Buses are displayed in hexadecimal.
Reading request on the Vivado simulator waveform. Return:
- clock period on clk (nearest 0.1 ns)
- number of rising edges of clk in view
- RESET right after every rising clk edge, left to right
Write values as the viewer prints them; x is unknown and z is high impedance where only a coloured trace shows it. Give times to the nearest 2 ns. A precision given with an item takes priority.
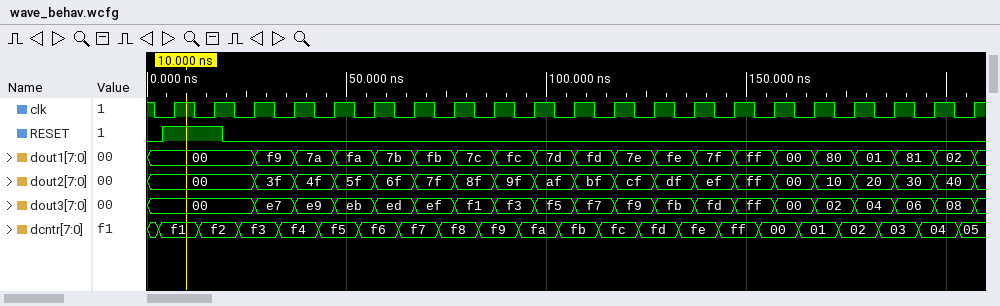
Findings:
10 ns
21
1 1 0 0 0 0 0 0 0 0 0 0 0 0 0 0 0 0 0 0 0
